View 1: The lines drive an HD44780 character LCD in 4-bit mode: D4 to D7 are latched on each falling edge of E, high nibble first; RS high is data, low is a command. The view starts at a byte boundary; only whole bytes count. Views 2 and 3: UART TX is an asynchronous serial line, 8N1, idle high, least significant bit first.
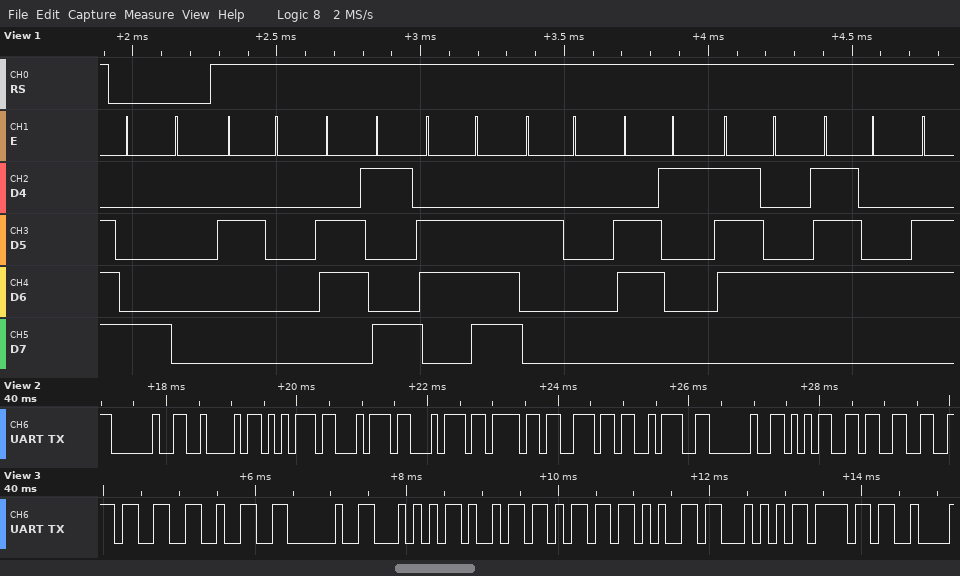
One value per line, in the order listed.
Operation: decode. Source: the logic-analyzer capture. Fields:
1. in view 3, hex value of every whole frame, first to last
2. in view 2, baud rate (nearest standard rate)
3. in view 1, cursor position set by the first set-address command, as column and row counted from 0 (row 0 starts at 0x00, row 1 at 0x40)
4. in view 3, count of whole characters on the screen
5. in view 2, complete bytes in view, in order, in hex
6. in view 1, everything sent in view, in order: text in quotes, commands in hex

33 32 20 54 69 6D 65 54 6F
9600 baud
column 0, row 0
9
0x20 0x42 0x75 0x74 0x74 0x6F 0x6E 0x3A 0x20 0x35 0x33
0x80 " in att"
